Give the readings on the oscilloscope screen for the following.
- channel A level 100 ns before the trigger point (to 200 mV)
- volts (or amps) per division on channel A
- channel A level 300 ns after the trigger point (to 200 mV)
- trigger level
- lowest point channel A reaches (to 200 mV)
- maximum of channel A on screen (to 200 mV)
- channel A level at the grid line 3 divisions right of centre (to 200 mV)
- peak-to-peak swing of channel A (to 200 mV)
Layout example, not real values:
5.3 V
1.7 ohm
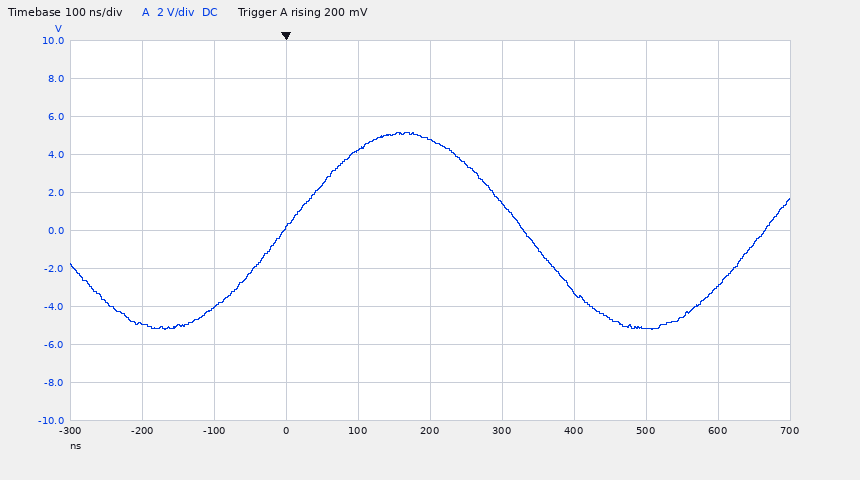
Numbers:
-4.0 V
2 V
1.4 V
200 mV
-5.2 V
5.2 V
-5.2 V
10.4 V
